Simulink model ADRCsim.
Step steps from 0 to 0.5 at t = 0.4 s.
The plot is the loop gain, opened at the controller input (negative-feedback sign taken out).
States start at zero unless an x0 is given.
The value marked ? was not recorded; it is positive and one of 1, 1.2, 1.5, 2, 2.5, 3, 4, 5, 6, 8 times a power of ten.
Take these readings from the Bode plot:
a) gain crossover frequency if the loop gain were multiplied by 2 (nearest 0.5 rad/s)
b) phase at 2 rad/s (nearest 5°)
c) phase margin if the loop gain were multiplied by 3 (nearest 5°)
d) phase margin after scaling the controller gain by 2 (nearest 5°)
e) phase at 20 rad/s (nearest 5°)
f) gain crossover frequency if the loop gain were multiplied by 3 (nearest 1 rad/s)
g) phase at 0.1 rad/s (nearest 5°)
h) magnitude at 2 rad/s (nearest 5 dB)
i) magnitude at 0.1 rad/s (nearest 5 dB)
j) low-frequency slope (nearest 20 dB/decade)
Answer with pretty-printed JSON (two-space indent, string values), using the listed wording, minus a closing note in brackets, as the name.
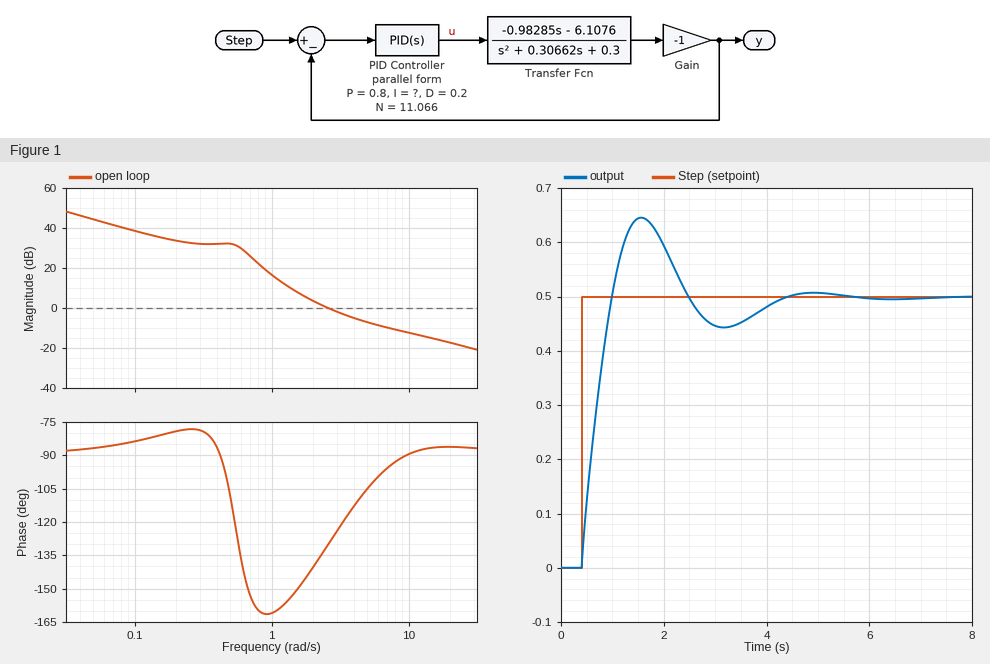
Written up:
{
  "gain crossover frequency if the loop gain were multiplied by 2": "4.5 rad/s",
  "phase at 2 rad/s": "-140°",
  "phase margin if the loop gain were multiplied by 3": "85°",
  "phase margin after scaling the controller gain by 2": "70°",
  "phase at 20 rad/s": "-85°",
  "gain crossover frequency if the loop gain were multiplied by 3": "7 rad/s",
  "phase at 0.1 rad/s": "-85°",
  "magnitude at 2 rad/s": "5 dB",
  "magnitude at 0.1 rad/s": "40 dB",
  "low-frequency slope": "-20 dB/decade"
}
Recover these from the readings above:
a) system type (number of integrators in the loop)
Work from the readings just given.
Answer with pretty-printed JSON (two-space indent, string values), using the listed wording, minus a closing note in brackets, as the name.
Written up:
{
  "system type": "1"
}
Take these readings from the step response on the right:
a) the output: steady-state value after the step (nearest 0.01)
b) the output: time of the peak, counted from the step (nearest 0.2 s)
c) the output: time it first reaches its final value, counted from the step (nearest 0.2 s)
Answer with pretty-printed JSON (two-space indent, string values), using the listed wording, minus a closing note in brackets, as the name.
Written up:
{
  "the output: steady-state value after the step": "0.50",
  "the output: time of the peak, counted from the step": "1.2 s",
  "the output: time it first reaches its final value, counted from the step": "0.6 s"
}
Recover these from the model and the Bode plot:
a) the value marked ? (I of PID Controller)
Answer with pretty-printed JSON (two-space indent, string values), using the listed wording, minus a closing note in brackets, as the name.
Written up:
{
  "the value marked ?": "0.4"
}
